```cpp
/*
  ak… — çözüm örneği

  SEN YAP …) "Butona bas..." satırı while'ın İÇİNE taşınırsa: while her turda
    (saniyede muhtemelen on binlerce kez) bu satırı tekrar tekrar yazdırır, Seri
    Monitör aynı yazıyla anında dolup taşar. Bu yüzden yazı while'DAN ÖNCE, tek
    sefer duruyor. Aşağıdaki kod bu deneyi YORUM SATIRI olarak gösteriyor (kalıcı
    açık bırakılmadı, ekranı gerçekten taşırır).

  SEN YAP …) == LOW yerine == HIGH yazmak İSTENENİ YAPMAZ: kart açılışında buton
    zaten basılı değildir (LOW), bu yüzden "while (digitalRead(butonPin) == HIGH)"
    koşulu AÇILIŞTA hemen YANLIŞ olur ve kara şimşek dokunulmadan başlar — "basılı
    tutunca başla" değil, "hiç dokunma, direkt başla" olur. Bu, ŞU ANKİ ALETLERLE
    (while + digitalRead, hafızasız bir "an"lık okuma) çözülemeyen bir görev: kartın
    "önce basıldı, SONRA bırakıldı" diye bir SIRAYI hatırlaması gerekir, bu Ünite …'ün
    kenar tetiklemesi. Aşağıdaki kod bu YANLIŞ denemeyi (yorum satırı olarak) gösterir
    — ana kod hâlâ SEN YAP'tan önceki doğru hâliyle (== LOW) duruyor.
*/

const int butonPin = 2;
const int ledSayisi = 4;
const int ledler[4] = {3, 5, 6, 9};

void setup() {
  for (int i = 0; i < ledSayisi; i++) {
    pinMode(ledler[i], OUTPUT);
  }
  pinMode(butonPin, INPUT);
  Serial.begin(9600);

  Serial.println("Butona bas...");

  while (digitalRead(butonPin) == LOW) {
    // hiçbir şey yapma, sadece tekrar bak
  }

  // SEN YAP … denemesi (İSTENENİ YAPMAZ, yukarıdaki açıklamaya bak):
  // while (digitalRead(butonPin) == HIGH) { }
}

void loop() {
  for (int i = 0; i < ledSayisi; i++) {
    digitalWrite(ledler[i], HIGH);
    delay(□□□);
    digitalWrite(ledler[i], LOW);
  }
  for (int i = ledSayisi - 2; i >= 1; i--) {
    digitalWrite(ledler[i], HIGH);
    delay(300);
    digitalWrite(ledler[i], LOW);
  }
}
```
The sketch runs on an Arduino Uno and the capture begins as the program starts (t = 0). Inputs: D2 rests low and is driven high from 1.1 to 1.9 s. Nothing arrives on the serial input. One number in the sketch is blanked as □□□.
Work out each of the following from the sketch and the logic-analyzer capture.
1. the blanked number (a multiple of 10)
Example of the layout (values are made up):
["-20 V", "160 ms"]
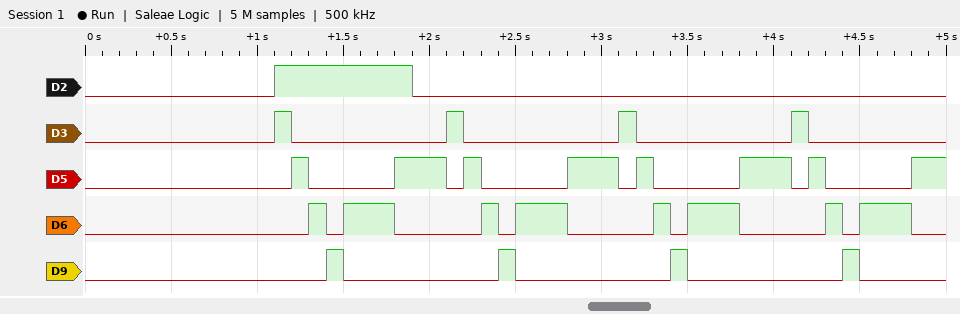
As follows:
["100"]
